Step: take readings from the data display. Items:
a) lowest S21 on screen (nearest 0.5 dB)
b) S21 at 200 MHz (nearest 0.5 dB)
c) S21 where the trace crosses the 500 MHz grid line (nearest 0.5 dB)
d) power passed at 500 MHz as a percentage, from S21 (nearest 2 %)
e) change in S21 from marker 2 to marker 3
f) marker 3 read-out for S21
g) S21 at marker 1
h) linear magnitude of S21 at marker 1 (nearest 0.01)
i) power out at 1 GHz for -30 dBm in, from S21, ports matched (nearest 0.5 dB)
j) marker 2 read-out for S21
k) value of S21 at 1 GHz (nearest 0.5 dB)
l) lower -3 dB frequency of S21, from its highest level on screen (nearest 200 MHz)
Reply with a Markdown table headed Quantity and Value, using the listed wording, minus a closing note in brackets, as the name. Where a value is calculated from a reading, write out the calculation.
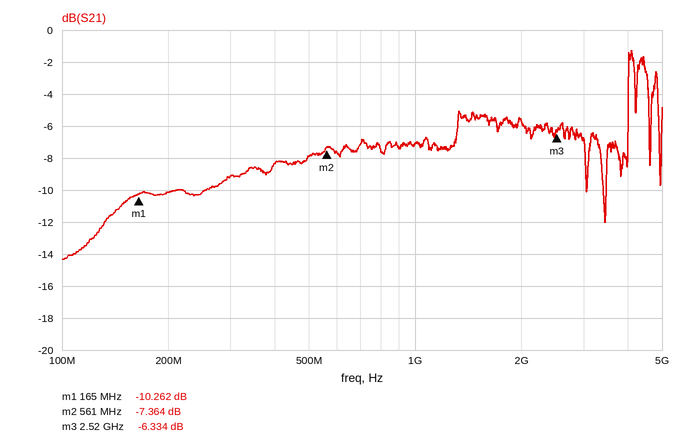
| Quantity | Value |
|---|---|
| lowest S21 on screen | -14.5 dB |
| S21 at 200 MHz | -10.0 dB |
| S21 where the trace crosses the 500 MHz grid line | -8.0 dB |
| power passed at 500 MHz as a percentage, from S21 | 10^(-8/10) ≈ 16 % |
| change in S21 from marker 2 to marker 3 | -6.334 − (-7.364) = 1.030 dB |
| marker 3 read-out for S21 | -6.334 dB |
| S21 at marker 1 | -10.262 dB |
| linear magnitude of S21 at marker 1 | 10^(-10.262/20) ≈ 0.31 |
| power out at 1 GHz for -30 dBm in, from S21, ports matched | -30 dBm + (-7.0 dB) = -37.0 dBm |
| marker 2 read-out for S21 | -7.364 dB |
| value of S21 at 1 GHz | -7.0 dB |
| lower -3 dB frequency of S21, from its highest level on screen | 4.0 GHz |
